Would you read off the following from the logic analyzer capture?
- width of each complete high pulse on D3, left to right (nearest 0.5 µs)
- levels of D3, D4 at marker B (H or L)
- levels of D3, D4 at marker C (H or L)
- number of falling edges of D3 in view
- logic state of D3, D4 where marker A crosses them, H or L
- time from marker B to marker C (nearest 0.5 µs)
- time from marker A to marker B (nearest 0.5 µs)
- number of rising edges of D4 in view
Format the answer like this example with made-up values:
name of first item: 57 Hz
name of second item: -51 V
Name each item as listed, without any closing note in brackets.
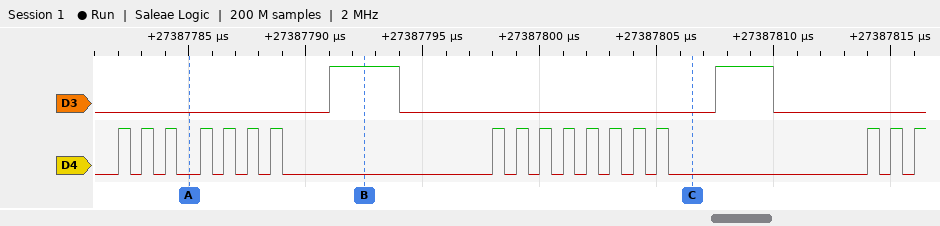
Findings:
width of each complete high pulse on D3, left to right: 3 µs, 2.5 µs
levels of D3, D4 at marker B: D3=H, D4=L
levels of D3, D4 at marker C: D3=L, D4=L
number of falling edges of D3 in view: 2
logic state of D3, D4 where marker A crosses them, H or L: D3=L, D4=L
time from marker B to marker C: 14 µs
time from marker A to marker B: 7.5 µs
number of rising edges of D4 in view: 18
